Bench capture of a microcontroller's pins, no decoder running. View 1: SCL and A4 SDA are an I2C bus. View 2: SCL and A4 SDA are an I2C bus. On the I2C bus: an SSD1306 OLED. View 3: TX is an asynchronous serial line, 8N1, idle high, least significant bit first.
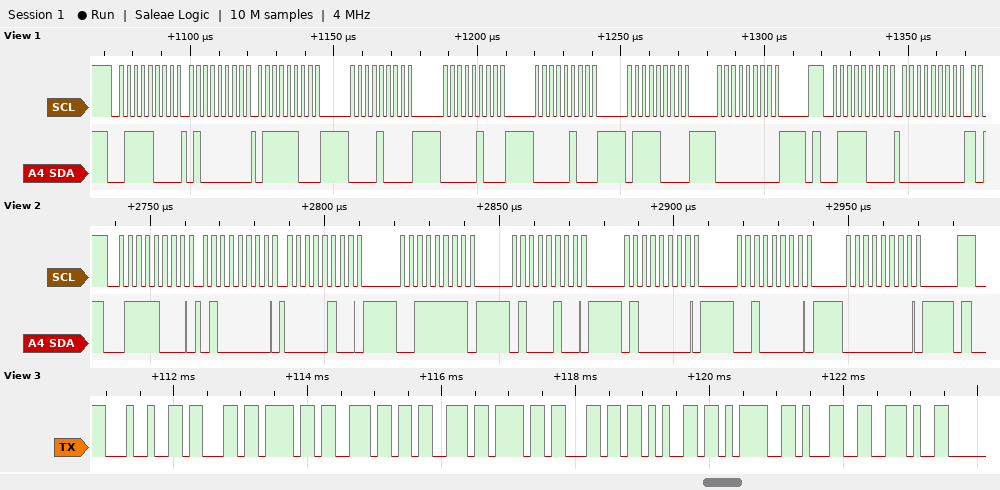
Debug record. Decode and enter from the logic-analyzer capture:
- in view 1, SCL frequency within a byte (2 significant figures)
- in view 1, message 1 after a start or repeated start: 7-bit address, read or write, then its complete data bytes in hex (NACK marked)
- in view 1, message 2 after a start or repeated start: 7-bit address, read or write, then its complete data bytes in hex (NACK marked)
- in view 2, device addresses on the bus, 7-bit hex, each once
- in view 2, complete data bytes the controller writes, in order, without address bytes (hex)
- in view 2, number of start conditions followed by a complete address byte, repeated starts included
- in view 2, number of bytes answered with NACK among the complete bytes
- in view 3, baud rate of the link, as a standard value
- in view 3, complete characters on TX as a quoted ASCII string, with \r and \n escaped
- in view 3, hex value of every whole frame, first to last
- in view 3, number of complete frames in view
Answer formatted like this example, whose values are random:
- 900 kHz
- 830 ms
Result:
- 400 kHz
- 0x3C write: 40 7C 08 04 04 78 00
- 0x3C write: 00
- 0x3C
- 40 04 3F 44 40 20 00
- 1
- 0
- 9600 baud
- "$console=1."
- 24 63 6F 6E 73 6F 6C 65 3D 31 2E
- 11
